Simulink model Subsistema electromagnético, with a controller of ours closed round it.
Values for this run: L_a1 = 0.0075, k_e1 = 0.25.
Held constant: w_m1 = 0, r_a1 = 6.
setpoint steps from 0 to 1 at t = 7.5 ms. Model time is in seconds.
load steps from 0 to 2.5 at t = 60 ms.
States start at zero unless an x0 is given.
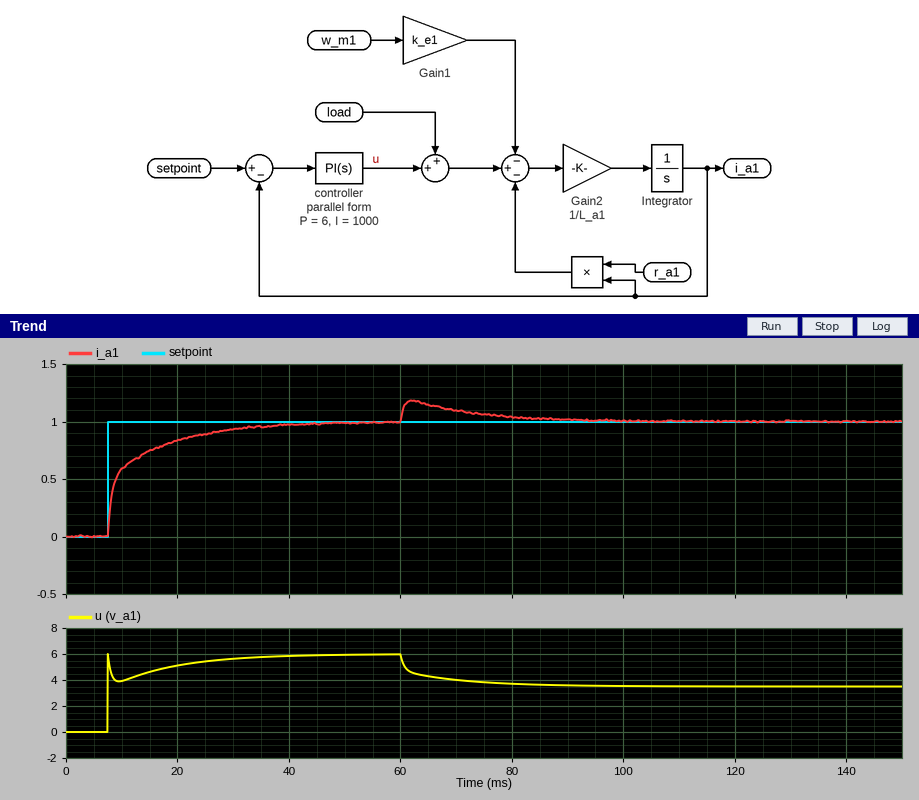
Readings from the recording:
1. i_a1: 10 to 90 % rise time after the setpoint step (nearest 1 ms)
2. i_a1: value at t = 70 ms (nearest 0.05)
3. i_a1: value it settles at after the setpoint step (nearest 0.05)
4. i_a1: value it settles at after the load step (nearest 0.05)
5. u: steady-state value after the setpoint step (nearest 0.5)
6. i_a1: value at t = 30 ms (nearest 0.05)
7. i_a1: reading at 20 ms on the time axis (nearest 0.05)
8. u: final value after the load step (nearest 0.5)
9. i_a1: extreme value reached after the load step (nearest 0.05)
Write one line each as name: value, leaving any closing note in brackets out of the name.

i_a1: 10 to 90 % rise time after the setpoint step: 18 ms
i_a1: value at t = 70 ms: 1.10
i_a1: value it settles at after the setpoint step: 1.00
i_a1: value it settles at after the load step: 1.00
u: steady-state value after the setpoint step: 6.0
i_a1: value at t = 30 ms: 0.95
i_a1: reading at 20 ms on the time axis: 0.85
u: final value after the load step: 3.5
i_a1: extreme value reached after the load step: 1.20
